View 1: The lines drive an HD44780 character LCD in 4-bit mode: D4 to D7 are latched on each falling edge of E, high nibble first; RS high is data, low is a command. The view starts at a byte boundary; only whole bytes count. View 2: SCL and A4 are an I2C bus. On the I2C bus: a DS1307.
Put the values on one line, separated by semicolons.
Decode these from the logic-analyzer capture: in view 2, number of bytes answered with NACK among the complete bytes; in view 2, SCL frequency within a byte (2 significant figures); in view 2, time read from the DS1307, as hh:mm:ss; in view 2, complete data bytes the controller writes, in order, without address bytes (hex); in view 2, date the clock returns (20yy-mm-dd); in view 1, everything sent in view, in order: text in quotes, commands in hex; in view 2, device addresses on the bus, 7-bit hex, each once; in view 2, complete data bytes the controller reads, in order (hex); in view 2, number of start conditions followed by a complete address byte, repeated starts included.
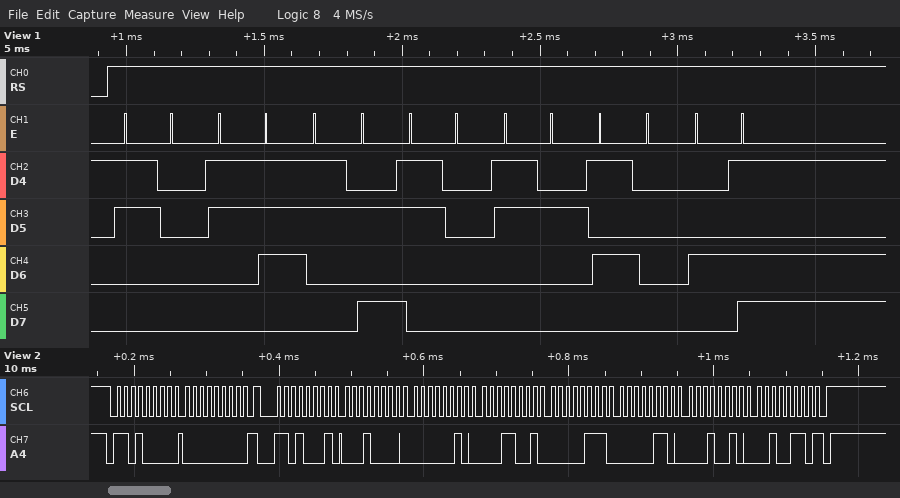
1; 100 kHz; 19:02:10; 00; 2026-12-06; "07:02PM"; 0x68; 10 02 19 07 06 12 26; 2
